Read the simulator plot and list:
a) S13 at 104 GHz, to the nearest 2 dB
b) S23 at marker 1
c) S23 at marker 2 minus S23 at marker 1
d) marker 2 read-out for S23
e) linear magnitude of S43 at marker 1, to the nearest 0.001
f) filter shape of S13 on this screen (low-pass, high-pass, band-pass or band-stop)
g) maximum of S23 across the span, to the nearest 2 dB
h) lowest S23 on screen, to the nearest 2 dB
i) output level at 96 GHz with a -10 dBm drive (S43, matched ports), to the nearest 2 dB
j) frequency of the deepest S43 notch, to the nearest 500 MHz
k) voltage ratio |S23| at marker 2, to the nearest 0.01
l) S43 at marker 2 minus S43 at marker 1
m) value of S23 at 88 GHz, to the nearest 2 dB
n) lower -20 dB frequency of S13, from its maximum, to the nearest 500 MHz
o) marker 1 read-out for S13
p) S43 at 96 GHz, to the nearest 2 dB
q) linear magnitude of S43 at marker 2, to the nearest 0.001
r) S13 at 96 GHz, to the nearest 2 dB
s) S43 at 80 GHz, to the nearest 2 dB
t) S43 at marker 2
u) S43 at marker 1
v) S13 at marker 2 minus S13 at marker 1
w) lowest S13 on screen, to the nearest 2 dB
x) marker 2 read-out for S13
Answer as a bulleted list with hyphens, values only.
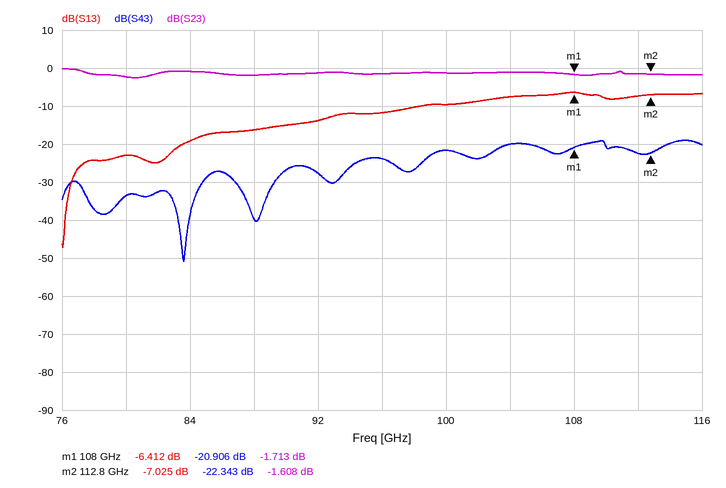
- -8 dB
- -1.713 dB
- 0.105 dB
- -1.608 dB
- 0.090
- high-pass
- 0 dB
- -2 dB
- -34 dBm
- 83.5 GHz
- 0.83
- -1.437 dB
- -2 dB
- 77.0 GHz
- -6.412 dB
- -24 dB
- 0.076
- -12 dB
- -34 dB
- -22.343 dB
- -20.906 dB
- -0.613 dB
- -48 dB
- -7.025 dB
